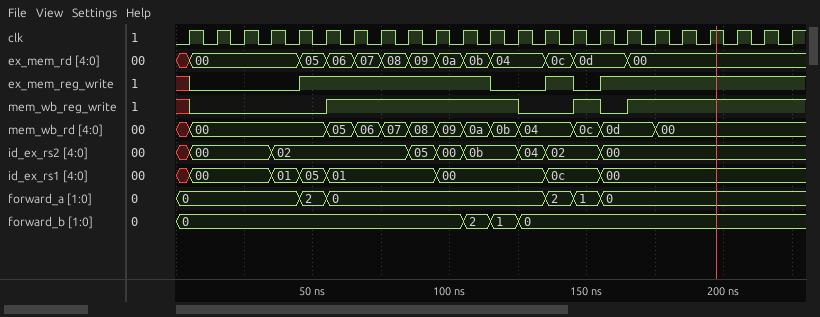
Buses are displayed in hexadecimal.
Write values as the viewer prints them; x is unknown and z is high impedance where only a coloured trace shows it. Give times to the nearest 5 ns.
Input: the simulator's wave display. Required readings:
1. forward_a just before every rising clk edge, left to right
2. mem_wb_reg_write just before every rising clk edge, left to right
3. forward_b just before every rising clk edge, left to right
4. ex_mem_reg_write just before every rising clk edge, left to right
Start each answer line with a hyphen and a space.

- 0, 0, 0, 0, 0, 2, 0, 0, 0, 0, 0, 0, 0, 0, 2, 1, 0, 0, 0, 0, 0, 0, 0
- x 0 0 0 0 0 1 1 1 1 1 1 1 0 0 1 0 1 1 1 1 1 1
- 0, 0, 0, 0, 0, 0, 0, 0, 0, 0, 0, 2, 1, 0, 0, 0, 0, 0, 0, 0, 0, 0, 0
- x 0 0 0 0 1 1 1 1 1 1 1 0 0 1 0 1 1 1 1 1 1 1
